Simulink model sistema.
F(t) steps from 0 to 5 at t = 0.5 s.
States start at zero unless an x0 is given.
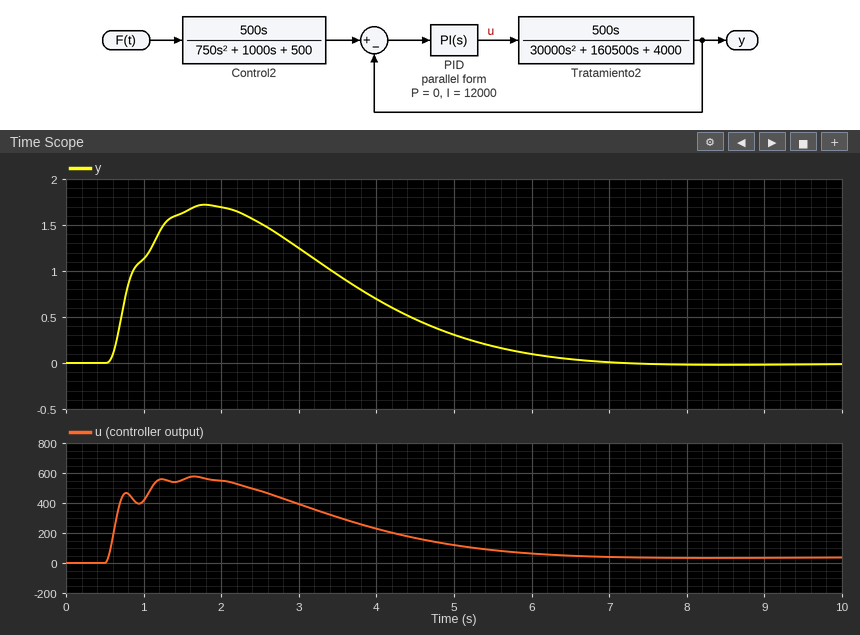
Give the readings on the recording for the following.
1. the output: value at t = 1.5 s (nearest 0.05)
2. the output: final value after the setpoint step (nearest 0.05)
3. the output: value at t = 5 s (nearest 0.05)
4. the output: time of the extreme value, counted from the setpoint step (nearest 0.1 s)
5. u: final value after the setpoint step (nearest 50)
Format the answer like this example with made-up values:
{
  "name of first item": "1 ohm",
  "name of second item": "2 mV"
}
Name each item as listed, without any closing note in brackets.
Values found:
{
  "the output: value at t = 1.5 s": "1.65",
  "the output: final value after the setpoint step": "0.00",
  "the output: value at t = 5 s": "0.30",
  "the output: time of the extreme value, counted from the setpoint step": "1.3 s",
  "u: final value after the setpoint step": "50"
}
